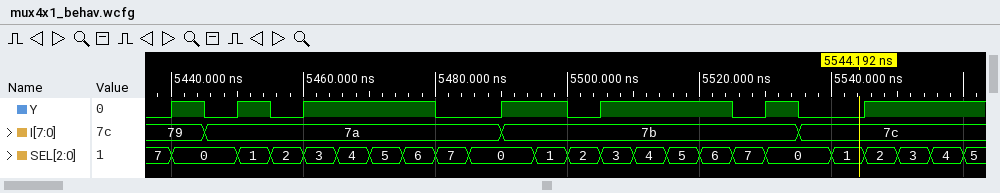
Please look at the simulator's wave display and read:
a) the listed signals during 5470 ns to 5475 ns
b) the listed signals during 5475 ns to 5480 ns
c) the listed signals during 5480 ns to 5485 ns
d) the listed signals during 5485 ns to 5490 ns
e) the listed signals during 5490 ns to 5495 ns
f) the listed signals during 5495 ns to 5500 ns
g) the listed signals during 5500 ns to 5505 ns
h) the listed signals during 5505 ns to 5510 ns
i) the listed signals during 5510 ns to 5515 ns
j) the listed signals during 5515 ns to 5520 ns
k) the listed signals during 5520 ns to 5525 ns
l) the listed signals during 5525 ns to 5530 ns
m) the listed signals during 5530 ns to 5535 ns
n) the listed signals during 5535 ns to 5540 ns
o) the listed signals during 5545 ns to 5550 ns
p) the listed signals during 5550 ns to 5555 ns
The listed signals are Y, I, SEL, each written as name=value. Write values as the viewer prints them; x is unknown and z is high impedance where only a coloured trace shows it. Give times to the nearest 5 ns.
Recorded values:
Y=1, I=7a, SEL=5
Y=1, I=7a, SEL=6
Y=0, I=7a, SEL=7
Y=0, I=7a, SEL=0
Y=1, I=7b, SEL=0
Y=1, I=7b, SEL=1
Y=0, I=7b, SEL=2
Y=1, I=7b, SEL=3
Y=1, I=7b, SEL=4
Y=1, I=7b, SEL=5
Y=1, I=7b, SEL=6
Y=0, I=7b, SEL=7
Y=1, I=7b, SEL=0
Y=0, I=7c, SEL=0
Y=1, I=7c, SEL=2
Y=1, I=7c, SEL=3
